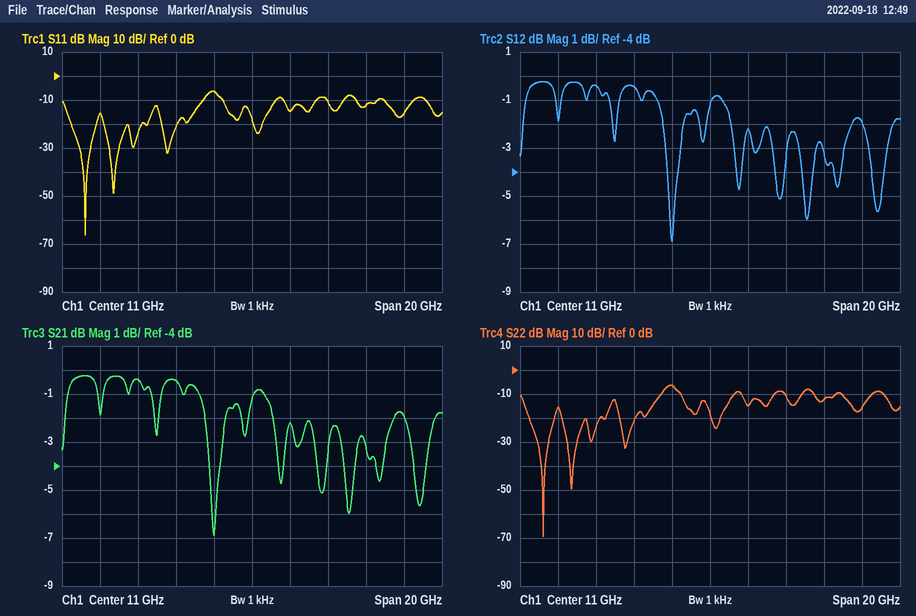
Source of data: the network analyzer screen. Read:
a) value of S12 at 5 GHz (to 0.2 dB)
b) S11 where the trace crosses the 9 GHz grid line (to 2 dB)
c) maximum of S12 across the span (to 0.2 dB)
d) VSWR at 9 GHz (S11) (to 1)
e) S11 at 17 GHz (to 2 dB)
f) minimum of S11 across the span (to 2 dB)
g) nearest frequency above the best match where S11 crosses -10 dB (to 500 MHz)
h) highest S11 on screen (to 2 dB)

-0.4 dB
-6 dB
-0.2 dB
3
-12 dB
-66 dB
8.5 GHz
-6 dB
